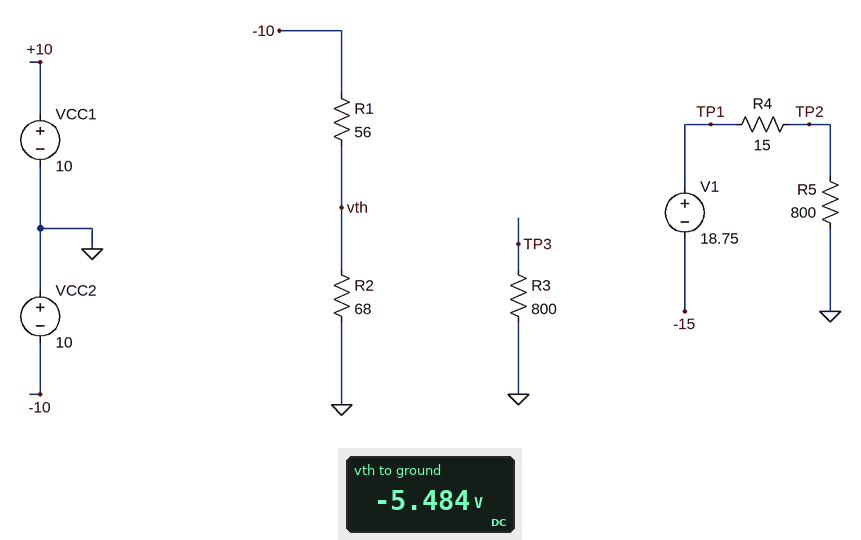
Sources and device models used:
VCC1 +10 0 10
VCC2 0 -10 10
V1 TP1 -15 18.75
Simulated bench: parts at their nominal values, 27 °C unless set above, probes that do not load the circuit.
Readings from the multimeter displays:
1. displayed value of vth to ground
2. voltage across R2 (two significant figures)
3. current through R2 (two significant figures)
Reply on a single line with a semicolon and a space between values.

-5.484 V; 5.5 V; 81 mA
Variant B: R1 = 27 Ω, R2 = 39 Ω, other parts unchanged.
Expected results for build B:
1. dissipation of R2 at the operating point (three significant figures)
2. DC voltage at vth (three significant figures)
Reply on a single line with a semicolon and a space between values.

895 mW; -5.91 V
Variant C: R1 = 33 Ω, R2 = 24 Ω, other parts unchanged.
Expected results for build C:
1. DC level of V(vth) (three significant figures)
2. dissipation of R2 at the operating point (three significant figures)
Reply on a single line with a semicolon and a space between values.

-4.21 V; 739 mW
